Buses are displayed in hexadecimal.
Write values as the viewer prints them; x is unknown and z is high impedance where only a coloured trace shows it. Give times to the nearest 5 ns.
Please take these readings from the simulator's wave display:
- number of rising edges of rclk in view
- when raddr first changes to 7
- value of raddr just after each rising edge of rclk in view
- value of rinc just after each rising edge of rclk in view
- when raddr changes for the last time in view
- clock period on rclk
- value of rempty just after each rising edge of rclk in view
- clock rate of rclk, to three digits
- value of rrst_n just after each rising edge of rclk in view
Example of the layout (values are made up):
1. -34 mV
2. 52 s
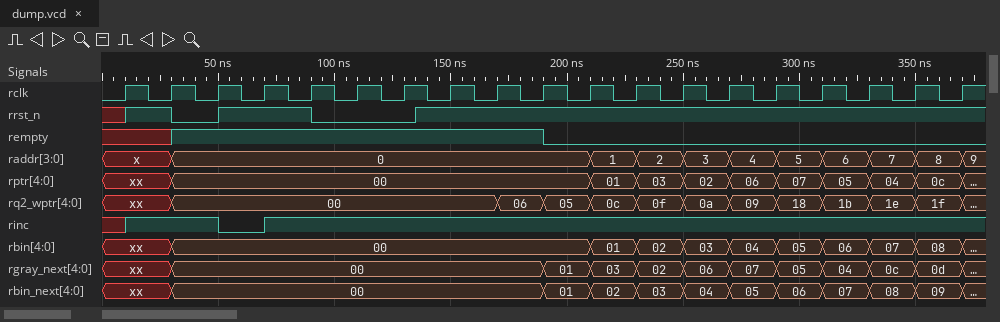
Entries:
1. 19
2. 330 ns
3. x, 0, 0, 0, 0, 0, 0, 0, 0, 0, 1, 2, 3, 4, 5, 6, 7, 8, 9
4. 1 1 0 1 1 1 1 1 1 1 1 1 1 1 1 1 1 1 1
5. 370 ns
6. 20 ns
7. x 1 1 1 1 1 1 1 1 0 0 0 0 0 0 0 0 0 0
8. 50.0 MHz
9. 1 0 1 1 0 0 0 1 1 1 1 1 1 1 1 1 1 1 1
